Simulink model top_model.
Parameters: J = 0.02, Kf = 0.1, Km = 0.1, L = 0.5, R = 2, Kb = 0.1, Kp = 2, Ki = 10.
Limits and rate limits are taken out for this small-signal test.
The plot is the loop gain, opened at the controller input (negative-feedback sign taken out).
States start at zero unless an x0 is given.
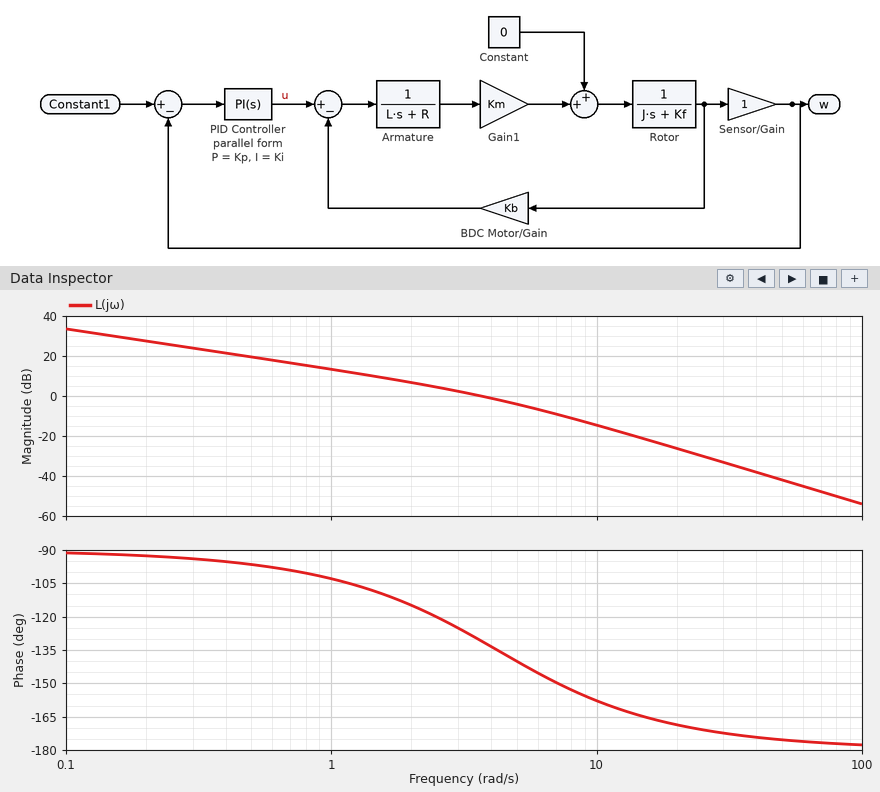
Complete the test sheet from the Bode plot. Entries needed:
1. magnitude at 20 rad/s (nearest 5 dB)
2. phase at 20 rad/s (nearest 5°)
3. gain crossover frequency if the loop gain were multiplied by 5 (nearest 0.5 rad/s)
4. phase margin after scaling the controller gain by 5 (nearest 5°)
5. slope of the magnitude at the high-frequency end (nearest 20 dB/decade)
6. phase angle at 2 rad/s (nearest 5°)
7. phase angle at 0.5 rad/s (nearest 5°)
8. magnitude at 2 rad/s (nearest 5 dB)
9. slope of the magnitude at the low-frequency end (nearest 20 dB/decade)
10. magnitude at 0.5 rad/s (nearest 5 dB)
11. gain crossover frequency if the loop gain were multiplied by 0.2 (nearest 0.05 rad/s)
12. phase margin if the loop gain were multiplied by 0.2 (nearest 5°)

-25 dB
-170°
9.5 rad/s
25°
-40 dB/decade
-115°
-95°
5 dB
-20 dB/decade
20 dB
0.95 rad/s
80°
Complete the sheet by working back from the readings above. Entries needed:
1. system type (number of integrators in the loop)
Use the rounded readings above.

1
